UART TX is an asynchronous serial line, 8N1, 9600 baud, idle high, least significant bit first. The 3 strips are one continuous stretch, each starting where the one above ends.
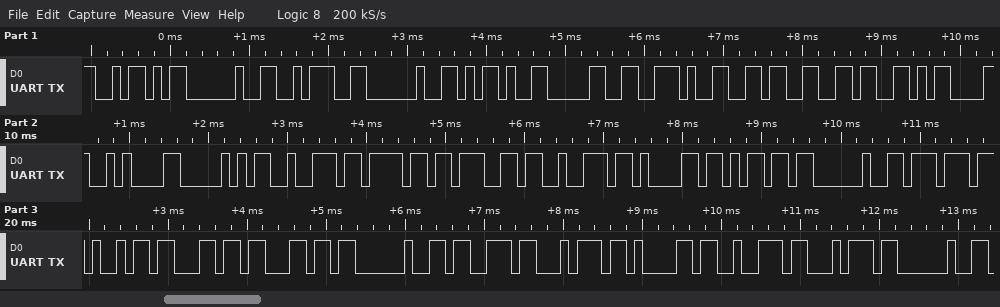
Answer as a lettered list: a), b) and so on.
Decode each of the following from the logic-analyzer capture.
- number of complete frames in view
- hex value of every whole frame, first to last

a) 30
b) 0x5A 0x20 0x3A 0x20 0x2D 0x30 0x2E 0x36 0x36 0x0D 0x0A 0x50 0x72 0x6F 0x67 0x72 0x61 0x6D 0x20 0x77 0x69 0x6C 0x6C 0x20 0x73 0x74 0x61 0x72 0x74 0x20
